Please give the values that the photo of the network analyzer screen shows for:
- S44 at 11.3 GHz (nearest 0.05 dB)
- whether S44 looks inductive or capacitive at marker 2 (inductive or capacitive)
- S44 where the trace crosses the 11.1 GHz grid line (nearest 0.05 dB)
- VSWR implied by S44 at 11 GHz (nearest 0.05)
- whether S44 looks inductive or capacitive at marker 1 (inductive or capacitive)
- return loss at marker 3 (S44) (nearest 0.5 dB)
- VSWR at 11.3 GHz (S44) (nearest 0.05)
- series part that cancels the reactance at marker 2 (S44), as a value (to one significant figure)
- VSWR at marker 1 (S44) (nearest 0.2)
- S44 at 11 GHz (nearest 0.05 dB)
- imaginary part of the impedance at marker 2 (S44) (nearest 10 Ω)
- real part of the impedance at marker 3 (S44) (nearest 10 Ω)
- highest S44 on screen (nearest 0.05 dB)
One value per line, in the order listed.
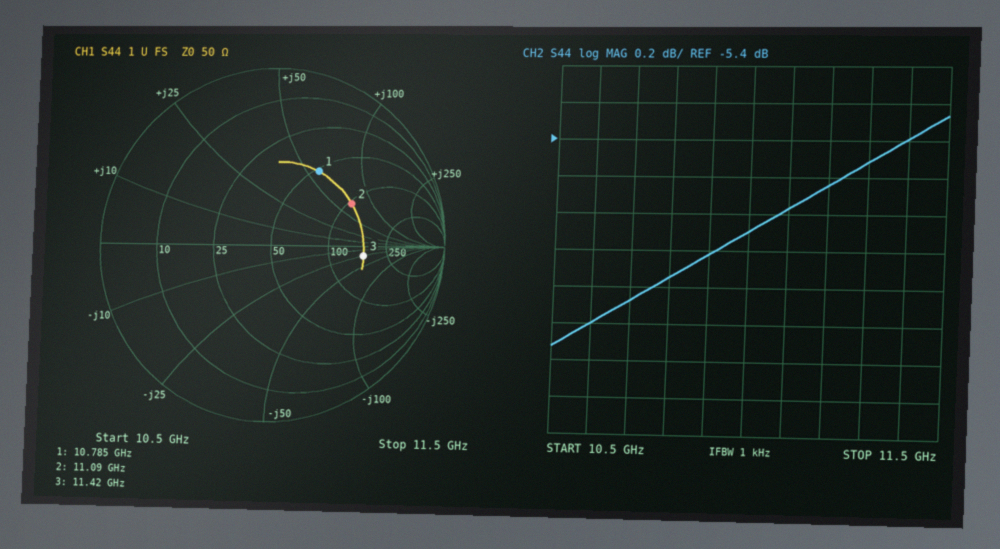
-5.50 dB
inductive
-5.75 dB
3.05
inductive
5.5 dB
3.25
200 fF
3.0
-5.90 dB
+70 Ω
160 Ω
-5.25 dB
